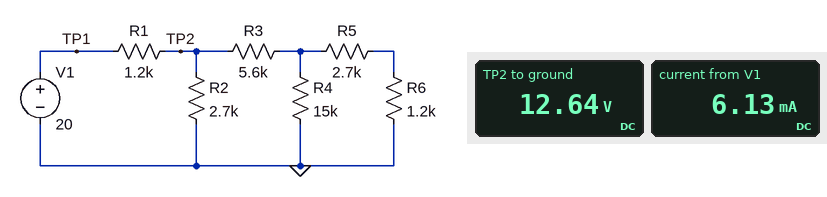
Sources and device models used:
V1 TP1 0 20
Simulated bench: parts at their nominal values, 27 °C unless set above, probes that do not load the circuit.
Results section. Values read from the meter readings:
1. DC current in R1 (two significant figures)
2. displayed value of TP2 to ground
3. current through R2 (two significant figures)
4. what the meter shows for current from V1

6.1 mA
12.64 V
4.7 mA
6.13 mA
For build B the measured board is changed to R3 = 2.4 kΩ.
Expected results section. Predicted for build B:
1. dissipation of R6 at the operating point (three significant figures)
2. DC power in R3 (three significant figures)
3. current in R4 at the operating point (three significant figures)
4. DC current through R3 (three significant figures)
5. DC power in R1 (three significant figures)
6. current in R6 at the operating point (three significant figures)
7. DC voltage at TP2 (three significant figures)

3.62 mW
11.5 mW
452 µA
2.19 mA
53.0 mW
1.74 mA
12.0 V
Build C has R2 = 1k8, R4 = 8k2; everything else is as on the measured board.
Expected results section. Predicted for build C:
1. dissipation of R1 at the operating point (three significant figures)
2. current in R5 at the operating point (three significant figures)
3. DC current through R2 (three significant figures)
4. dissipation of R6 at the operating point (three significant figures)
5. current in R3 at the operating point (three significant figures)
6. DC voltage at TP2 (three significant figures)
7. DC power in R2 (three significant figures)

67.0 mW
907 µA
6.13 mA
988 µW
1.34 mA
11.0 V
67.7 mW
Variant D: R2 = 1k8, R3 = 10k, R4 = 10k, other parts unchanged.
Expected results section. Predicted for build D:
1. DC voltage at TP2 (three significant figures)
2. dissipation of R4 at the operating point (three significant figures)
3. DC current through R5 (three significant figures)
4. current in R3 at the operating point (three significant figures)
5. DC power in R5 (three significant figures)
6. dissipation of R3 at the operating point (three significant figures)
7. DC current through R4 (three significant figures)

11.4 V
620 µW
638 µA
887 µA
1.10 mW
7.87 mW
249 µA
